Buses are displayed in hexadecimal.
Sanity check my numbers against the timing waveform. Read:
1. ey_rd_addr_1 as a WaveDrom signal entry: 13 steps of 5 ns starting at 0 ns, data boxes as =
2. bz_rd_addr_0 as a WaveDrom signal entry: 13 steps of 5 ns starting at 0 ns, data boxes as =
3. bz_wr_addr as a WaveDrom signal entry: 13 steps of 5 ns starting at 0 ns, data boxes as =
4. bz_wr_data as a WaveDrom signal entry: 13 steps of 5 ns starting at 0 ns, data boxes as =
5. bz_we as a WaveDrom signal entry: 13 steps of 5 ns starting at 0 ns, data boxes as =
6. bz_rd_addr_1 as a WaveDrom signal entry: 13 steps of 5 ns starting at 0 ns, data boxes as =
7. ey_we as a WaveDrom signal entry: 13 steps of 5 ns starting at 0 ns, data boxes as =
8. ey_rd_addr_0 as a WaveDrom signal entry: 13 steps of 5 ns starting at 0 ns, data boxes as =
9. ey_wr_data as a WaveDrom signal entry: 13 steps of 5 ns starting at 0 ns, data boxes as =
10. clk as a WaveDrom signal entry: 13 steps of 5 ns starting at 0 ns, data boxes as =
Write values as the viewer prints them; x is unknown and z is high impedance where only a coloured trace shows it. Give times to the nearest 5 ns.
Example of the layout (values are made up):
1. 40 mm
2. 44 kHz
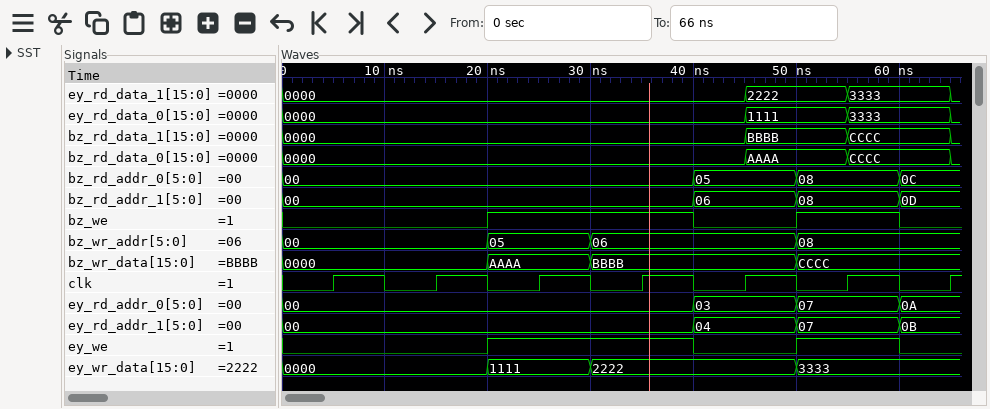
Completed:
1. {name: 'ey_rd_addr_1', wave: '=.......=.=.=', data: '00 04 07 0B'}
2. {name: 'bz_rd_addr_0', wave: '=.......=.=.=', data: '00 05 08 0C'}
3. {name: 'bz_wr_addr', wave: '=...=.=...=..', data: '00 05 06 08'}
4. {name: 'bz_wr_data', wave: '=...=.=...=..', data: '0000 AAAA BBBB CCCC'}
5. {name: 'bz_we', wave: '0...1...0.1.0'}
6. {name: 'bz_rd_addr_1', wave: '=.......=.=.=', data: '00 06 08 0D'}
7. {name: 'ey_we', wave: '0...1...0.1.0'}
8. {name: 'ey_rd_addr_0', wave: '=.......=.=.=', data: '00 03 07 0A'}
9. {name: 'ey_wr_data', wave: '=...=.=...=..', data: '0000 1111 2222 3333'}
10. {name: 'clk', wave: '0101010101010'}
